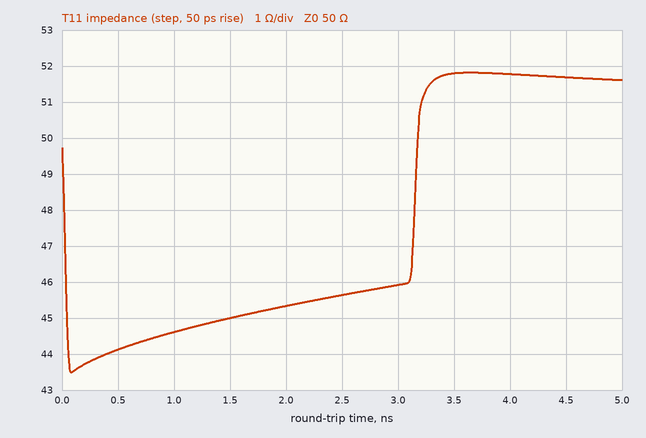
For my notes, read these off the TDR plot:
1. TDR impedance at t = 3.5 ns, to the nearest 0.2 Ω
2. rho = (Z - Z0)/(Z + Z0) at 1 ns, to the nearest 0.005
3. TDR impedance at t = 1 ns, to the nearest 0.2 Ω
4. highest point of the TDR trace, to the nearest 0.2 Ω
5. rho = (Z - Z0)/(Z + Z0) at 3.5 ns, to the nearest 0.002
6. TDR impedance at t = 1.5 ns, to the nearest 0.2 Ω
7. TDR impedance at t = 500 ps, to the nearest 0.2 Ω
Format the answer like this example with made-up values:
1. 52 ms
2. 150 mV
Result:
1. 51.8 Ω
2. -0.055
3. 44.6 Ω
4. 51.8 Ω
5. +0.018
6. 45.0 Ω
7. 44.2 Ω
